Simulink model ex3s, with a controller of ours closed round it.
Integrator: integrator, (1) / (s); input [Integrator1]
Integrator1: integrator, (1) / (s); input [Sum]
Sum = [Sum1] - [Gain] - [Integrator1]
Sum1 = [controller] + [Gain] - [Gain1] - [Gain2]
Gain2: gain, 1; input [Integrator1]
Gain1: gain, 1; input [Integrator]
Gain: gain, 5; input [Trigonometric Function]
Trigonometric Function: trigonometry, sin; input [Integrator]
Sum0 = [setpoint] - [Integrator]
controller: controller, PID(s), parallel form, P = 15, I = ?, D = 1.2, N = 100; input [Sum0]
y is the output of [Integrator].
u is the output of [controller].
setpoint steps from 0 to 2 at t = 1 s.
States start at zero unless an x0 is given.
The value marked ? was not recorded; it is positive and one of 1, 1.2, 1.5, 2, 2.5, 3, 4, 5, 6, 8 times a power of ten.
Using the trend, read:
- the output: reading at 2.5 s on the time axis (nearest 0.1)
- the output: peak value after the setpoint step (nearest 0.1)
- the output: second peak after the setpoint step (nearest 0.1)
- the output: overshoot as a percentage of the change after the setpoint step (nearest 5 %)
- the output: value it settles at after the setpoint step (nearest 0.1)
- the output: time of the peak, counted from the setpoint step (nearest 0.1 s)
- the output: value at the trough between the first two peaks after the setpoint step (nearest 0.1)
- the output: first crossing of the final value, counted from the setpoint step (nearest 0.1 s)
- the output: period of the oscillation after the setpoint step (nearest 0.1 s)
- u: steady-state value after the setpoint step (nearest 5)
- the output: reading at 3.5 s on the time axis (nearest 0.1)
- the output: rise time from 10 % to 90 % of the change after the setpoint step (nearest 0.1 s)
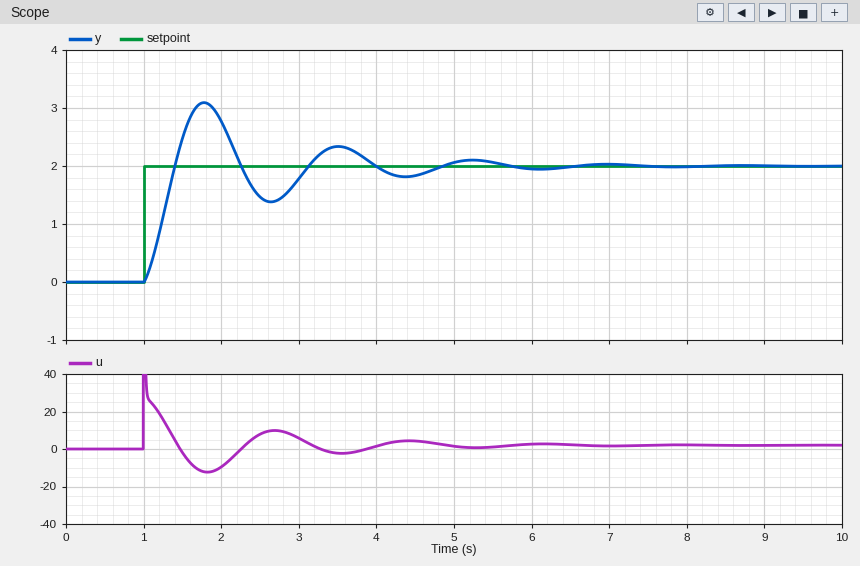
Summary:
1.5
3.1
2.3
55 %
2.0
0.8 s
1.4
0.4 s
1.7 s
0
2.3
0.3 s
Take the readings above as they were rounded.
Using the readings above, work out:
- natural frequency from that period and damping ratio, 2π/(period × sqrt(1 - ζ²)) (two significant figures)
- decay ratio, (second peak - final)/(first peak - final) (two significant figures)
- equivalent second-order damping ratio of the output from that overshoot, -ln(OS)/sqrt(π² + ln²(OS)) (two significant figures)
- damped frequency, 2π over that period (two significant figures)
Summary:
3.8 rad/s
0.27
0.19
3.7 rad/s
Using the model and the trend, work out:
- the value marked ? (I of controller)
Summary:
25
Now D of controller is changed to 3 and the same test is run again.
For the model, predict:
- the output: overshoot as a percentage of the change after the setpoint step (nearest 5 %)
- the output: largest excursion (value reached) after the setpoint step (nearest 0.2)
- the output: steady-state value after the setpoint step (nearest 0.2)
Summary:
30 %
2.6
2.0
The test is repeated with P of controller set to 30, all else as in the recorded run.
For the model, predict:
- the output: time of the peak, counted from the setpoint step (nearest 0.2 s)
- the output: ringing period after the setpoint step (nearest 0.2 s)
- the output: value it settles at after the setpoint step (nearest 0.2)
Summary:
0.6 s
1.2 s
2.0
